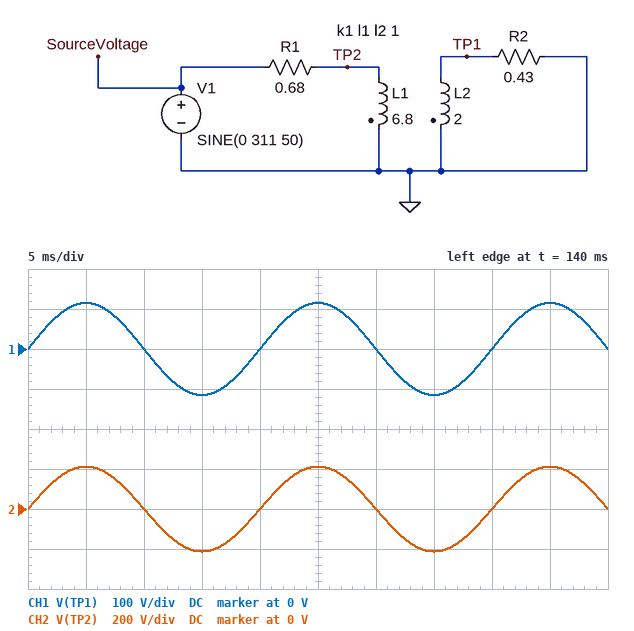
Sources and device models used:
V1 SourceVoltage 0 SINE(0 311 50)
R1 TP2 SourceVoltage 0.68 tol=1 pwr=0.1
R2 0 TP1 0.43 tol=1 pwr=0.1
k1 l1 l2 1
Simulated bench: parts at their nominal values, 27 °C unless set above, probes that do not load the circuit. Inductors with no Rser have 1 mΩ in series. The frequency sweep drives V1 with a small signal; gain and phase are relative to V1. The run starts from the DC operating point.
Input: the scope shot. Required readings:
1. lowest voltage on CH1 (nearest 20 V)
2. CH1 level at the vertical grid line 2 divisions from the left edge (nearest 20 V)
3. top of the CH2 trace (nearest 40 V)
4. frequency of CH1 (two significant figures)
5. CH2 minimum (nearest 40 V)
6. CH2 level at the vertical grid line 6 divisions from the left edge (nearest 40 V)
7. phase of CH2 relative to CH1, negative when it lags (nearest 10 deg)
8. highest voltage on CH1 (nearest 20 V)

-120 V
0 V
200 V
50 Hz
-200 V
0 V
0 deg
120 V
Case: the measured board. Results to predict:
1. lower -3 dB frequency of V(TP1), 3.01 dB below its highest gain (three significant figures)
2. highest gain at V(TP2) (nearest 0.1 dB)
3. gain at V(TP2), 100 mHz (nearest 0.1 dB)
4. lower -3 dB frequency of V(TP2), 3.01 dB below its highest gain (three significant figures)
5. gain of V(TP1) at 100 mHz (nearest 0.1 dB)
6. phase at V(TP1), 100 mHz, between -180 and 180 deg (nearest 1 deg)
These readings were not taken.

10.9 mHz
-3.3 dB
-3.4 dB
10.9 mHz
-8.7 dB
6 deg
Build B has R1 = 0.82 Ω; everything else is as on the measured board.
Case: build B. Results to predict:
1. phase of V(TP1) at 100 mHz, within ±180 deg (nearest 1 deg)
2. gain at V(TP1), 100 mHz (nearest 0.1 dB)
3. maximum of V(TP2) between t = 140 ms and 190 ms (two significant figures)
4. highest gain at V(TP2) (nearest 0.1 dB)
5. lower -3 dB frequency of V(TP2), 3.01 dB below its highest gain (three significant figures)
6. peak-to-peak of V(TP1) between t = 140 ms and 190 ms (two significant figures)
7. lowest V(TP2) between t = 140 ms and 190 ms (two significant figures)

7 deg
-9.3 dB
200 V
-3.9 dB
12.3 mHz
220 V
-200 V
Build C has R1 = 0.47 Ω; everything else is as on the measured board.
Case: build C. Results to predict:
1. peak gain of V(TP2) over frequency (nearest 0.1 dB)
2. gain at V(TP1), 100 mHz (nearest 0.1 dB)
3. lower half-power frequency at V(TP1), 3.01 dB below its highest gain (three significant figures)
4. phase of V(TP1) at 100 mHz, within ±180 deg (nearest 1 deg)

-2.4 dB
-7.8 dB
8.34 mHz
5 deg
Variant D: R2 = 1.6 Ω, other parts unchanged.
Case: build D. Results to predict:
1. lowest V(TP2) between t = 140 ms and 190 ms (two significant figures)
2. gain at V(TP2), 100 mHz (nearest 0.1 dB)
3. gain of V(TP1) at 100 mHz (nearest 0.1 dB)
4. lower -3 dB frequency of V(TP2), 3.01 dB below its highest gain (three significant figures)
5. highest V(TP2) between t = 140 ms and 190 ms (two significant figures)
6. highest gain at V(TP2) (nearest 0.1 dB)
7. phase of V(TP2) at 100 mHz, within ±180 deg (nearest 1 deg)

-280 V
-1.1 dB
-6.4 dB
14.2 mHz
280 V
-1.0 dB
8 deg
